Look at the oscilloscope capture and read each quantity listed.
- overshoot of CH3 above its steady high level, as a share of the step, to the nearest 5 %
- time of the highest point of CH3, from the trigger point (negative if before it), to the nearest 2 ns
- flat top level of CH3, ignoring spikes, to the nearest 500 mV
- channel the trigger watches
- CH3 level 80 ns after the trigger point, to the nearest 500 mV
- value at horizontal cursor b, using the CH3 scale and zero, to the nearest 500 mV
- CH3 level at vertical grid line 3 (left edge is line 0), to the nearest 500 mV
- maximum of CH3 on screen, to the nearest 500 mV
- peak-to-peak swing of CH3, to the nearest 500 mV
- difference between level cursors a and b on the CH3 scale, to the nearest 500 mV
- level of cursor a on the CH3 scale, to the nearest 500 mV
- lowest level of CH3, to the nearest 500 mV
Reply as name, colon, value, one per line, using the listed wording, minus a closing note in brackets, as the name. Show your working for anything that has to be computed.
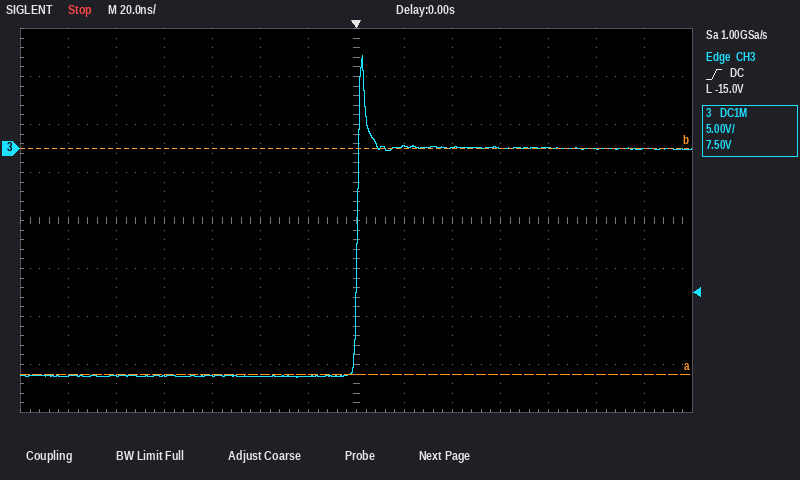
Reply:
overshoot of CH3 above its steady high level, as a share of the step, to the nearest 5 %: 40 %
time of the highest point of CH3, from the trigger point (negative if before it), to the nearest 2 ns: +2 ns
flat top level of CH3, ignoring spikes, to the nearest 500 mV: 0.0 V
channel the trigger watches: CH3
CH3 level 80 ns after the trigger point, to the nearest 500 mV: 0.0 V
value at horizontal cursor b, using the CH3 scale and zero, to the nearest 500 mV: 0.0 V
CH3 level at vertical grid line 3 (left edge is line 0), to the nearest 500 mV: -23.5 V
maximum of CH3 on screen, to the nearest 500 mV: 9.5 V
peak-to-peak swing of CH3, to the nearest 500 mV: 9.5 V − (-24.0 V) = 33.5 V
difference between level cursors a and b on the CH3 scale, to the nearest 500 mV: 23.5 V
level of cursor a on the CH3 scale, to the nearest 500 mV: -23.5 V
lowest level of CH3, to the nearest 500 mV: -24.0 V
